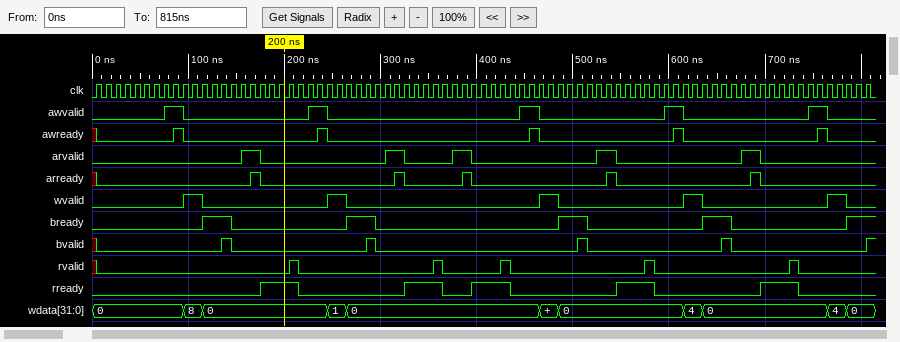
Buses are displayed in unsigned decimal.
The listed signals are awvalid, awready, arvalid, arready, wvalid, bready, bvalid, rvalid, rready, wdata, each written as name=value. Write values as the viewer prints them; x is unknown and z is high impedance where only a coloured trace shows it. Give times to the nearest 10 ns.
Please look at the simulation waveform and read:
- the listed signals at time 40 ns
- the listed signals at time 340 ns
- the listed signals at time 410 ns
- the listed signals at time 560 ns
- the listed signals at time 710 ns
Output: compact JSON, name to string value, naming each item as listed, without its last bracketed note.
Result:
{"the listed signals at time 40 ns": "awvalid=0, awready=0, arvalid=0, arready=0, wvalid=0, bready=0, bvalid=0, rvalid=0, rready=0, wdata=0", "the listed signals at time 340 ns": "awvalid=0, awready=0, arvalid=0, arready=0, wvalid=0, bready=0, bvalid=0, rvalid=0, rready=1, wdata=0", "the listed signals at time 410 ns": "awvalid=0, awready=0, arvalid=0, arready=0, wvalid=0, bready=0, bvalid=0, rvalid=0, rready=1, wdata=0", "the listed signals at time 560 ns": "awvalid=0, awready=0, arvalid=0, arready=0, wvalid=0, bready=0, bvalid=0, rvalid=0, rready=1, wdata=0", "the listed signals at time 710 ns": "awvalid=0, awready=0, arvalid=0, arready=0, wvalid=0, bready=0, bvalid=0, rvalid=0, rready=1, wdata=0"}
